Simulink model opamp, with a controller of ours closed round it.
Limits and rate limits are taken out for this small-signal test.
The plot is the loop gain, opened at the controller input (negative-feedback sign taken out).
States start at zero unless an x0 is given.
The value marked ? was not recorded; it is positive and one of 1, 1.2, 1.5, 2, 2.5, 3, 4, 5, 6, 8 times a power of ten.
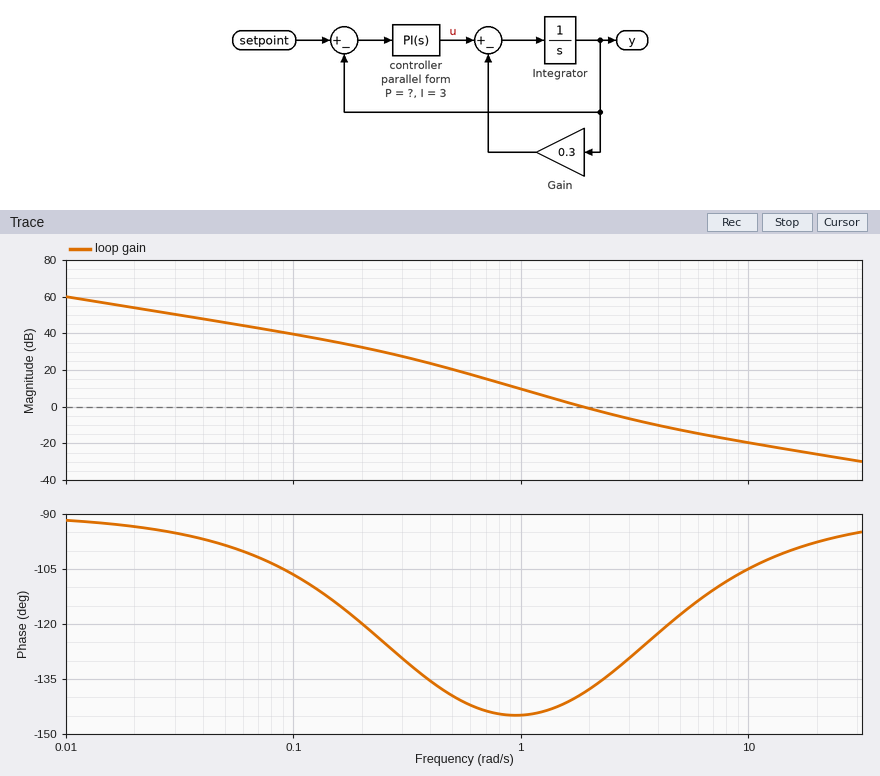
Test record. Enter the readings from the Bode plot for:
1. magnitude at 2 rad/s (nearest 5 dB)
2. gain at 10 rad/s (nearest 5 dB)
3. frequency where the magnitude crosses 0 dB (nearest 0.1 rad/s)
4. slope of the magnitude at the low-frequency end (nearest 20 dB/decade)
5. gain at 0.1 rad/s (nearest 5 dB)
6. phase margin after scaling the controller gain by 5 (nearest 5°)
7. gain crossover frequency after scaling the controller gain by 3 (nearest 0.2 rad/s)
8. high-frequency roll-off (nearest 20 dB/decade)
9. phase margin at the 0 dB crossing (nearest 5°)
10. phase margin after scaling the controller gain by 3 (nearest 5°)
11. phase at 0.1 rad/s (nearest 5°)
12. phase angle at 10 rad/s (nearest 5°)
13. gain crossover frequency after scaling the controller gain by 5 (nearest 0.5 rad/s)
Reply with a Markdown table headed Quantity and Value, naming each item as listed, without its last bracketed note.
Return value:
| Quantity | Value |
|---|---|
| magnitude at 2 rad/s | 0 dB |
| gain at 10 rad/s | -20 dB |
| frequency where the magnitude crosses 0 dB | 1.9 rad/s |
| slope of the magnitude at the low-frequency end | -20 dB/decade |
| gain at 0.1 rad/s | 40 dB |
| phase margin after scaling the controller gain by 5 | 65° |
| gain crossover frequency after scaling the controller gain by 3 | 3.8 rad/s |
| high-frequency roll-off | -20 dB/decade |
| phase margin at the 0 dB crossing | 40° |
| phase margin after scaling the controller gain by 3 | 55° |
| phase at 0.1 rad/s | -105° |
| phase angle at 10 rad/s | -105° |
| gain crossover frequency after scaling the controller gain by 5 | 5.5 rad/s |
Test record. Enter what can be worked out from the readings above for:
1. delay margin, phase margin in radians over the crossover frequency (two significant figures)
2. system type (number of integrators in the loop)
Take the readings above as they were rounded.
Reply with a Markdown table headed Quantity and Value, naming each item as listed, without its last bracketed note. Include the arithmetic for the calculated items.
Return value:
| Quantity | Value |
|---|---|
| delay margin, phase margin in radians over the crossover frequency | 40 × π / 180 / 1.9 = 0.37 s |
| system type | 1 |
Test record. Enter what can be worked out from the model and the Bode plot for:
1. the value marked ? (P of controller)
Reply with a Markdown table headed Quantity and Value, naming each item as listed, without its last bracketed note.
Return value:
| Quantity | Value |
|---|---|
| the value marked ? | 1 |
